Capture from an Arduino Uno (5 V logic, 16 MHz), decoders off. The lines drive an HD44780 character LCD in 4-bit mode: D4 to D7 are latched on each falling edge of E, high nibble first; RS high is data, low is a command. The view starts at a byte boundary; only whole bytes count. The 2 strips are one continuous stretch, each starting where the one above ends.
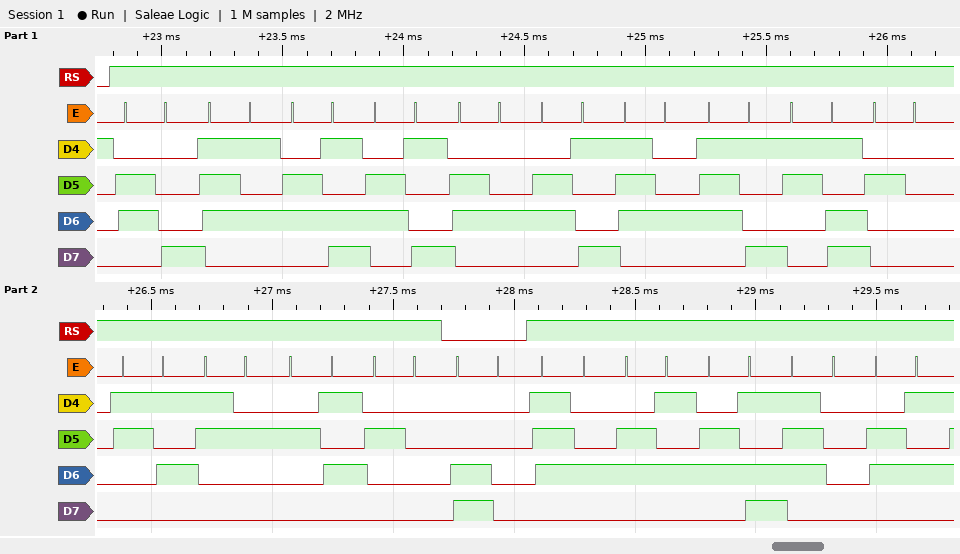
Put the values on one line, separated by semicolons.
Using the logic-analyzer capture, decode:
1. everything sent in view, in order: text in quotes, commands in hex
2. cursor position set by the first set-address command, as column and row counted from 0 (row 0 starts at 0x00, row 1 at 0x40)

"humidity= 52% " 0xC0 "tempe"; column 0, row 1
